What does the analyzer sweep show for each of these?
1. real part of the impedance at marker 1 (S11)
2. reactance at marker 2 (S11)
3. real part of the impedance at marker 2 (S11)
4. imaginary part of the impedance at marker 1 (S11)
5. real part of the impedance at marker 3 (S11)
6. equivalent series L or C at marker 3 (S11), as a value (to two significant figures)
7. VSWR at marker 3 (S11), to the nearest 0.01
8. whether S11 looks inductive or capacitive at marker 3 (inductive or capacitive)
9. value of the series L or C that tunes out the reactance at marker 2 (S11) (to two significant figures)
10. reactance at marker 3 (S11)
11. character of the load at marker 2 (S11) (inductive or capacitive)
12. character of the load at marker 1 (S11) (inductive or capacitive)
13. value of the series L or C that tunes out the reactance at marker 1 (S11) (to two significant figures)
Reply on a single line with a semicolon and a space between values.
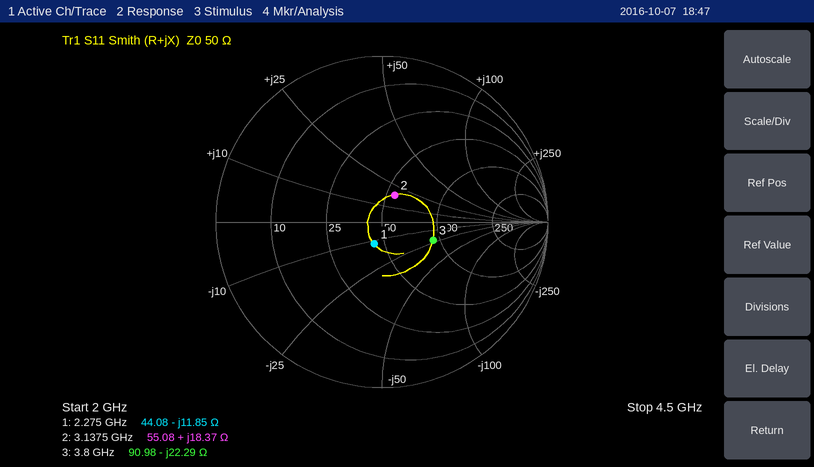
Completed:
44.08 Ω; +18.37 Ω; 55.08 Ω; -11.85 Ω; 90.98 Ω; 1.9 pF; 1.97; capacitive; 2.8 pF; -22.29 Ω; inductive; capacitive; 830 pH
